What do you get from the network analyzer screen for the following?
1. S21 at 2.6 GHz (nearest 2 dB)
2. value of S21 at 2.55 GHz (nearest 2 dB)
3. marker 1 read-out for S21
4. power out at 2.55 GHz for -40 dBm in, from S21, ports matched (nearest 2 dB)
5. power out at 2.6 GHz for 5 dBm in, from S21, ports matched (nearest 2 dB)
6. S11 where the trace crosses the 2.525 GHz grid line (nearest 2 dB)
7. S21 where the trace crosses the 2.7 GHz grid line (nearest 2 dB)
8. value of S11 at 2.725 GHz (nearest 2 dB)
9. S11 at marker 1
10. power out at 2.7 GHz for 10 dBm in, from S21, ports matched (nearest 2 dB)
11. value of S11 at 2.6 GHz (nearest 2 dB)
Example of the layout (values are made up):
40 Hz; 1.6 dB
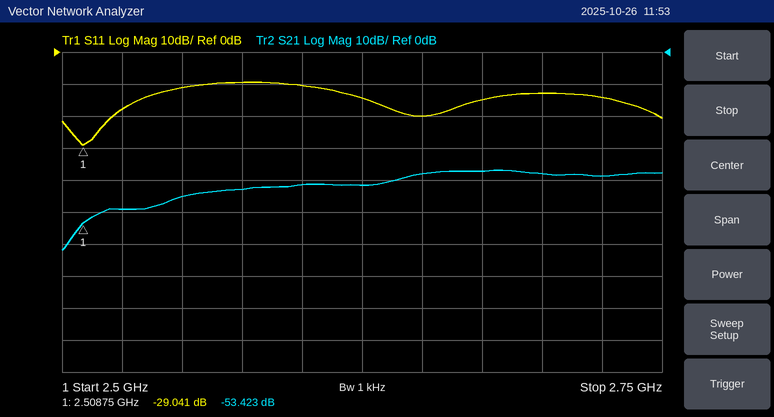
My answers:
-42 dB; -46 dB; -53.423 dB; -86 dBm; -36 dBm; -18 dB; -38 dB; -14 dB; -29.041 dB; -28 dBm; -10 dB
